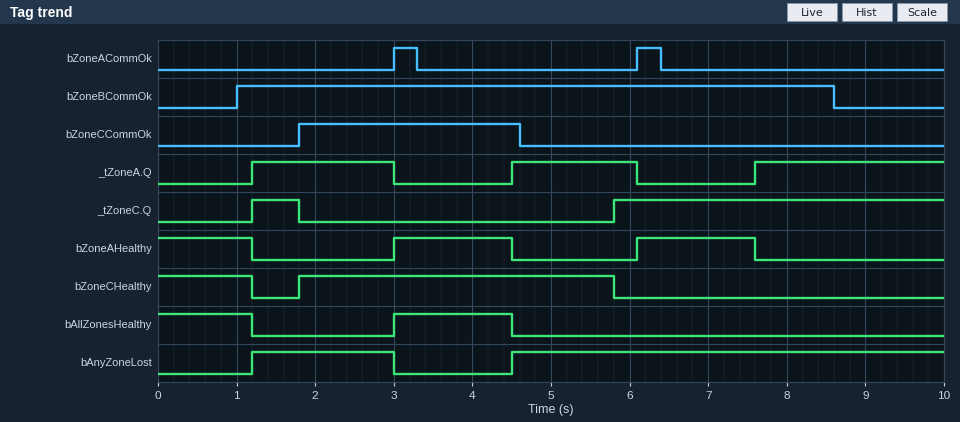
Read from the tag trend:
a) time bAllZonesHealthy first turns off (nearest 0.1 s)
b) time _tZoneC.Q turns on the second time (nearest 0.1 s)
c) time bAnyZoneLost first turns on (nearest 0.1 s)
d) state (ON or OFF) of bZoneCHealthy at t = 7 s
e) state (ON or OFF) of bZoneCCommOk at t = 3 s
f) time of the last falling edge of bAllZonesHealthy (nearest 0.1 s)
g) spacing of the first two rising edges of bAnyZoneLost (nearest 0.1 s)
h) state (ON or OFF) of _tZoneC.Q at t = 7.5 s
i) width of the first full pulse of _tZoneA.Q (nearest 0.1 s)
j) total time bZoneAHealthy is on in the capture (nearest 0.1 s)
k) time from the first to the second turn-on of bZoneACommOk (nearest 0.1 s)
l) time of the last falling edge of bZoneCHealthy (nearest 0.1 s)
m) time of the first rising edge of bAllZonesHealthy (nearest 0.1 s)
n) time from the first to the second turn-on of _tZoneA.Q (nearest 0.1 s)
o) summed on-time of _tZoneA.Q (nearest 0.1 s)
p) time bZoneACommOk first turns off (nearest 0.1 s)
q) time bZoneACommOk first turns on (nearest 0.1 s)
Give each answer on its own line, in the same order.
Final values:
1.2 s
5.8 s
1.2 s
OFF
ON
4.5 s
3.3 s
ON
1.8 s
4.2 s
3.1 s
5.8 s
3.0 s
3.3 s
5.8 s
3.3 s
3.0 s
